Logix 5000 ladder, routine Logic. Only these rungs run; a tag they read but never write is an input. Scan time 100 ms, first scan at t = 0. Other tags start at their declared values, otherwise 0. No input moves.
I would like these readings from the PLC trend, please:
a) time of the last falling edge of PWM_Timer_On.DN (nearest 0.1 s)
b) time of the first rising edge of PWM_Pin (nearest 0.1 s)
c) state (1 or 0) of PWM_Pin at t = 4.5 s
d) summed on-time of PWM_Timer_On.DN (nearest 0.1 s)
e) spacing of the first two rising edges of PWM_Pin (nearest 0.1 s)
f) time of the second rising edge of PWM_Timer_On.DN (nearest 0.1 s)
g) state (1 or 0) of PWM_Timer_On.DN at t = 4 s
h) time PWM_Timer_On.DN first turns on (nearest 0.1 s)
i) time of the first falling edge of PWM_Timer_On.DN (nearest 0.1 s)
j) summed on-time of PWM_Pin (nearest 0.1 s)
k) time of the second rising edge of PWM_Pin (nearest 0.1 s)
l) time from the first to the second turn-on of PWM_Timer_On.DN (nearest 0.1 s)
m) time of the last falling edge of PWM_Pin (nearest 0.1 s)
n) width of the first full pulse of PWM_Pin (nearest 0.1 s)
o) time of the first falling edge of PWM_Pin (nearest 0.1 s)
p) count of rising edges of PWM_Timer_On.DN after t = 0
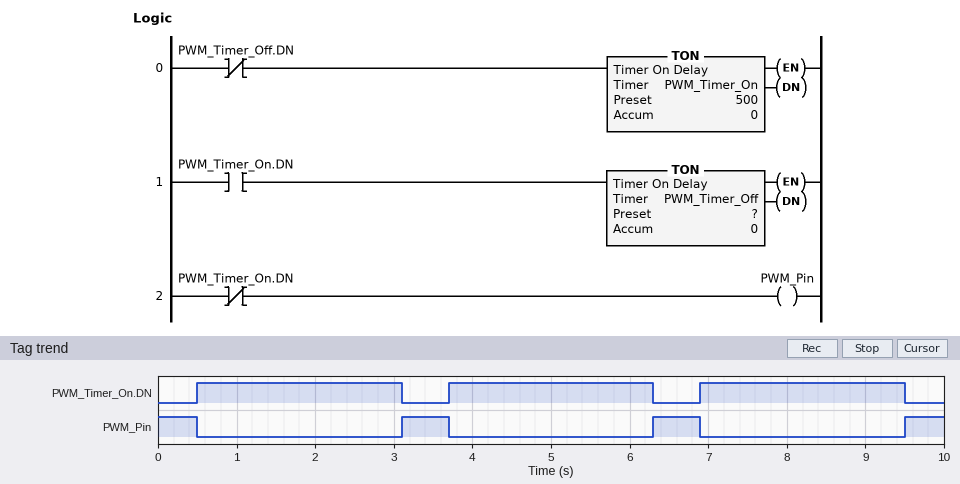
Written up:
9.5 s
3.1 s
0
7.8 s
3.2 s
3.7 s
1
0.5 s
3.1 s
2.2 s
6.3 s
3.2 s
6.9 s
0.6 s
0.5 s
3
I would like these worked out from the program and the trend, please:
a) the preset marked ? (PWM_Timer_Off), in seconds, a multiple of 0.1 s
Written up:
2.5 s
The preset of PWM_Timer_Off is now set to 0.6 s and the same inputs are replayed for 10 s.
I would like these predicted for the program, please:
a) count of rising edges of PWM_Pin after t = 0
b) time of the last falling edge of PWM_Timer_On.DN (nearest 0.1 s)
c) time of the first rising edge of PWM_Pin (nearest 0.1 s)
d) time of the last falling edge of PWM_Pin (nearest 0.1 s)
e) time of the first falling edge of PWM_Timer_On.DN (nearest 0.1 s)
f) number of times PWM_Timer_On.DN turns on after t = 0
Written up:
7
9.0 s
1.2 s
9.6 s
1.2 s
8
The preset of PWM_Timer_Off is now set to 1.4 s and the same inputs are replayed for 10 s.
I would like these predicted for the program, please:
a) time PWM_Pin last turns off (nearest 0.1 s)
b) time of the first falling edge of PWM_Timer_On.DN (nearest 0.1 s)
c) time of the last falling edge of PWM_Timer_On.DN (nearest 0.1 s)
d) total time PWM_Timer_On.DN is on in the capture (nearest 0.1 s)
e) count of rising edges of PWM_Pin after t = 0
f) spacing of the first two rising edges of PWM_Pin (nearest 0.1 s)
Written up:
8.9 s
2.0 s
8.3 s
7.1 s
4
2.1 s
